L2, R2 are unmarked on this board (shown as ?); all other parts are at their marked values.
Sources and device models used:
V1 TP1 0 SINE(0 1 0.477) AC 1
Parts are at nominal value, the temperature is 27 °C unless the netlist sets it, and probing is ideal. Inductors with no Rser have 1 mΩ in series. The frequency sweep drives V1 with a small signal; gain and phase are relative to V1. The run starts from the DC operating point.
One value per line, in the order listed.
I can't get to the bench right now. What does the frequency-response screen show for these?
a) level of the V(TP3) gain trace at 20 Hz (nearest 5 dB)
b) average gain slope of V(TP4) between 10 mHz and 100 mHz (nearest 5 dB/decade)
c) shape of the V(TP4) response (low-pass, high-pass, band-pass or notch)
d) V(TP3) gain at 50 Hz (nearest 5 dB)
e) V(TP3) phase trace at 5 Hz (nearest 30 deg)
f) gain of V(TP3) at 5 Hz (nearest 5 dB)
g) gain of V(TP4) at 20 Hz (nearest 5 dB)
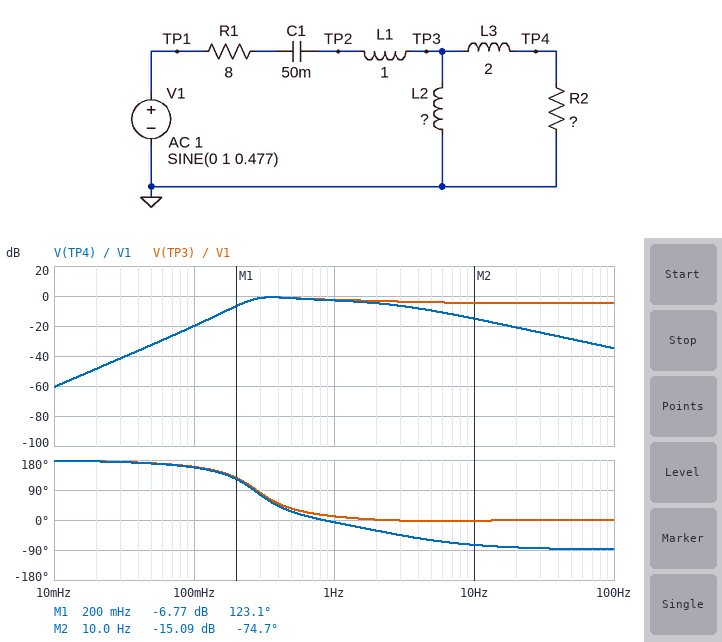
-5 dB
40 dB/decade
band-pass
-5 dB
0 deg
-5 dB
-20 dB
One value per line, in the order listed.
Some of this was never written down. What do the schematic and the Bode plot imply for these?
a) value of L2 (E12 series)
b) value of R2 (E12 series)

4.7 H
39 Ω
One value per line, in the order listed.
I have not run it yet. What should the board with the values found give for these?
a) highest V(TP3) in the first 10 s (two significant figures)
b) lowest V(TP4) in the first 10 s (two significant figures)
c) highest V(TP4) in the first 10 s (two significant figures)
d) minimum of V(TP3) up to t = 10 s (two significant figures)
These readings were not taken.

950 mV
-870 mV
940 mV
-880 mV
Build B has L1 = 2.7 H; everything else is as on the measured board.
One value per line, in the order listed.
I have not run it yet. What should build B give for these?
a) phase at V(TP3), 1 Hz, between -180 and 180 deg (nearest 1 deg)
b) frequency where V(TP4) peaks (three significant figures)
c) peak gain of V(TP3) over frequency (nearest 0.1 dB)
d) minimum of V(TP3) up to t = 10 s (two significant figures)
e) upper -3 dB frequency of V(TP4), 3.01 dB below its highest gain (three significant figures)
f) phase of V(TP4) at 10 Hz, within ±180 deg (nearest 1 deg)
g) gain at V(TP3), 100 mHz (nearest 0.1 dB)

0 deg
299 mHz
-1.6 dB
-720 mV
788 mHz
-79 deg
-19.7 dB
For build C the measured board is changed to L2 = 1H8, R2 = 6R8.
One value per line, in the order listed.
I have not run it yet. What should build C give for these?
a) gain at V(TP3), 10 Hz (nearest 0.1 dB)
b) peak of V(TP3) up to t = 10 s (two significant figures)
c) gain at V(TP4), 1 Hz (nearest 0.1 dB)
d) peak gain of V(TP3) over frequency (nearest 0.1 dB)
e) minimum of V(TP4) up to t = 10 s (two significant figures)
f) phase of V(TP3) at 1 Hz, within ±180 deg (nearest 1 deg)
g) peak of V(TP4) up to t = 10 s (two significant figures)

-6.3 dB
410 mV
-12.7 dB
-6.2 dB
-300 mV
32 deg
310 mV
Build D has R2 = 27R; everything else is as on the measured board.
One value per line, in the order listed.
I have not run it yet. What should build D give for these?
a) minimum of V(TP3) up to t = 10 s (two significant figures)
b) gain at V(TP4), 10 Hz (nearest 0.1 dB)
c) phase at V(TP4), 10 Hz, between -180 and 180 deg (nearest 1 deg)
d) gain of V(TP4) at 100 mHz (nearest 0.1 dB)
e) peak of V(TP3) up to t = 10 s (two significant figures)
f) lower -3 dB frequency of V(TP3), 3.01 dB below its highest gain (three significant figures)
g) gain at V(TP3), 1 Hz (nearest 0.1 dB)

-810 mV
-18.2 dB
-78 deg
-20.1 dB
870 mV
234 mHz
-3.1 dB
